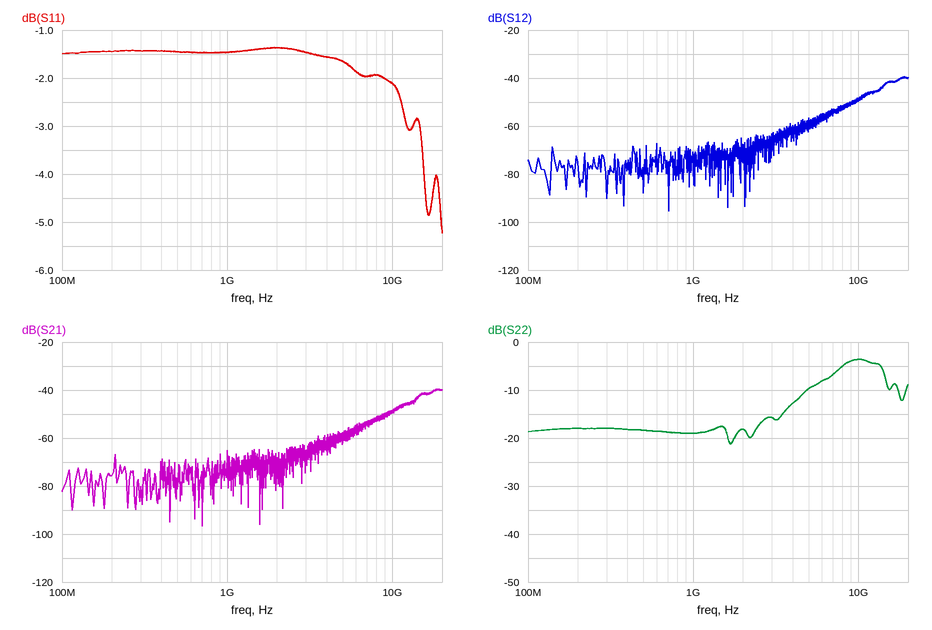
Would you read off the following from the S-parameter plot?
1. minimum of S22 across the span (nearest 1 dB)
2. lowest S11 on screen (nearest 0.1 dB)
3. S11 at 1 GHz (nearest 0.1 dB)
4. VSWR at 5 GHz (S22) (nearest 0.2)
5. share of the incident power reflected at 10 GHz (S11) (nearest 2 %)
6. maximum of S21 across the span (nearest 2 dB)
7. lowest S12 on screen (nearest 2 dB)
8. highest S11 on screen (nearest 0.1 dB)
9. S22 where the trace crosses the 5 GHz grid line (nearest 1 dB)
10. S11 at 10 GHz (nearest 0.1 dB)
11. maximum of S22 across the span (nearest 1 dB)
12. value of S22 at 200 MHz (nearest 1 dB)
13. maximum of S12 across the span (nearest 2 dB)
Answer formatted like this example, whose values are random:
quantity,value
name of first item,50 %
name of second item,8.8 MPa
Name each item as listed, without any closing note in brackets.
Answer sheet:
quantity,value
minimum of S22 across the span,-21 dB
lowest S11 on screen,-5.2 dB
S11 at 1 GHz,-1.5 dB
VSWR at 5 GHz (S22),2.0
share of the incident power reflected at 10 GHz (S11),62 %
maximum of S21 across the span,-40 dB
lowest S12 on screen,-96 dB
highest S11 on screen,-1.4 dB
S22 where the trace crosses the 5 GHz grid line,-10 dB
S11 at 10 GHz,-2.1 dB
maximum of S22 across the span,-4 dB
value of S22 at 200 MHz,-18 dB
maximum of S12 across the span,-40 dB
